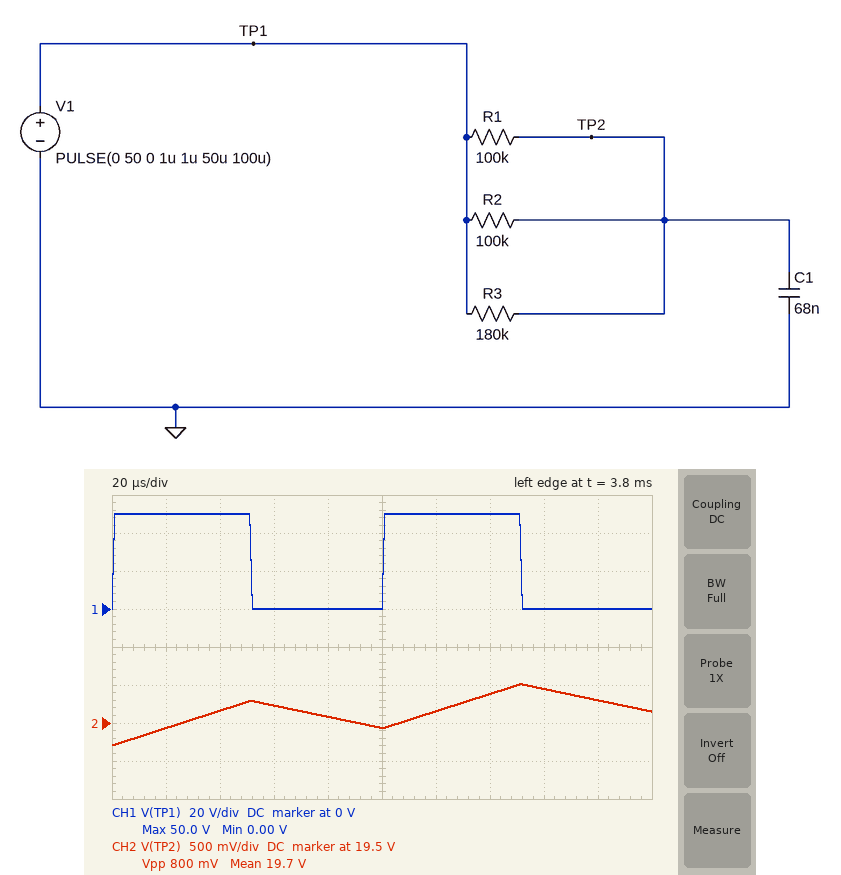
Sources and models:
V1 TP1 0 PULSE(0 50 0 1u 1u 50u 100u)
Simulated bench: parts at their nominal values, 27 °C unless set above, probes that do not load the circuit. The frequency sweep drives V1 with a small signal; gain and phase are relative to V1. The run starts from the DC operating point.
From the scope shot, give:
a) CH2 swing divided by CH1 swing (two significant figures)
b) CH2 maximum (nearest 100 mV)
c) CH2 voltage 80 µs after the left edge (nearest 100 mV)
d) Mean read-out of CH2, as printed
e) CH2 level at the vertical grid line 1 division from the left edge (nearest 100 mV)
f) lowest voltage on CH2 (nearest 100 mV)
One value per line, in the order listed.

0.016
20.0 V
19.6 V
19.7 V
19.4 V
19.2 V
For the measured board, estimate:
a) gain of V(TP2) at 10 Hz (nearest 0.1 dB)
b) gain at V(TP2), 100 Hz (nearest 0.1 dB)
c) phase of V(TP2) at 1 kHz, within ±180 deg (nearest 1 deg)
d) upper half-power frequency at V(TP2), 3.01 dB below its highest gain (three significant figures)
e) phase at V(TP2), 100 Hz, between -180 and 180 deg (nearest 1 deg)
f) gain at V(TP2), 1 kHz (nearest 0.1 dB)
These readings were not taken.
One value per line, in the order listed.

-0.1 dB
-5.8 dB
-87 deg
59.8 Hz
-59 deg
-24.5 dB
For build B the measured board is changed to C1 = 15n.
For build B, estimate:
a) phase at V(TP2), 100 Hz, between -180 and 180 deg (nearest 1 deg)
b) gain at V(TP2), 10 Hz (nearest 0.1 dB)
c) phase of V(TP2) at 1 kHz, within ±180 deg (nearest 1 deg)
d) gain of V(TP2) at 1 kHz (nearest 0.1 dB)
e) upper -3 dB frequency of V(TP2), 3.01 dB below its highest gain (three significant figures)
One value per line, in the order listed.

-20 deg
0 dB
-75 deg
-11.6 dB
271 Hz
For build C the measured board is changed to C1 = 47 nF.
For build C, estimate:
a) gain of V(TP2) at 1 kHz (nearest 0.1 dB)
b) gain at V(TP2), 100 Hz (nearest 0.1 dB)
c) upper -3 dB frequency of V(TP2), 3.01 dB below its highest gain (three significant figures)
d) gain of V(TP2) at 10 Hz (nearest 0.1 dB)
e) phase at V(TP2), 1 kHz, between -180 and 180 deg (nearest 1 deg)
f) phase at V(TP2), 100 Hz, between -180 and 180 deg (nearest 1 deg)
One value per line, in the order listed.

-21.3 dB
-3.7 dB
86.5 Hz
-0.1 dB
-85 deg
-49 deg
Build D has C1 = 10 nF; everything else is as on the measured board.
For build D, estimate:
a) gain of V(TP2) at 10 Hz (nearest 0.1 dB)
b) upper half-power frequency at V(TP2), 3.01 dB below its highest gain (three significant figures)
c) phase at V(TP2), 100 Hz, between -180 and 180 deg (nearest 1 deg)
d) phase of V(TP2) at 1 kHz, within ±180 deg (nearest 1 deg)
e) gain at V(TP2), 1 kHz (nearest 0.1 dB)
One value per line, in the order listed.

0 dB
407 Hz
-14 deg
-68 deg
-8.5 dB
